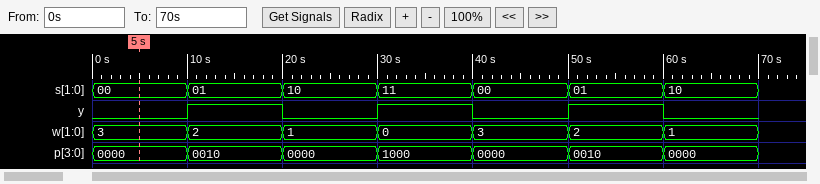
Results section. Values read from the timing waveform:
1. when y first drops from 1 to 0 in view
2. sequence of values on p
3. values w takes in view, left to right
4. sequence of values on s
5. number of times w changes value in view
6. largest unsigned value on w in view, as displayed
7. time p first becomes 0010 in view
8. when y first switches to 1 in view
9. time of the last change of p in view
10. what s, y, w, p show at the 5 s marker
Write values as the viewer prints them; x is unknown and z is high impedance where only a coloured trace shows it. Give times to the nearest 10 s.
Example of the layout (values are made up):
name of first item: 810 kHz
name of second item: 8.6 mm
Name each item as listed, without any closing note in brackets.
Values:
when y first drops from 1 to 0 in view: 20 s
sequence of values on p: 0000, 0010, 0000, 1000, 0000, 0010, 0000
values w takes in view, left to right: 3, 2, 1, 0, 3, 2, 1
sequence of values on s: 00, 01, 10, 11, 00, 01, 10
number of times w changes value in view: 6
largest unsigned value on w in view, as displayed: 3
time p first becomes 0010 in view: 10 s
when y first switches to 1 in view: 10 s
time of the last change of p in view: 60 s
what s, y, w, p show at the 5 s marker: s=00, y=0, w=3, p=0000
